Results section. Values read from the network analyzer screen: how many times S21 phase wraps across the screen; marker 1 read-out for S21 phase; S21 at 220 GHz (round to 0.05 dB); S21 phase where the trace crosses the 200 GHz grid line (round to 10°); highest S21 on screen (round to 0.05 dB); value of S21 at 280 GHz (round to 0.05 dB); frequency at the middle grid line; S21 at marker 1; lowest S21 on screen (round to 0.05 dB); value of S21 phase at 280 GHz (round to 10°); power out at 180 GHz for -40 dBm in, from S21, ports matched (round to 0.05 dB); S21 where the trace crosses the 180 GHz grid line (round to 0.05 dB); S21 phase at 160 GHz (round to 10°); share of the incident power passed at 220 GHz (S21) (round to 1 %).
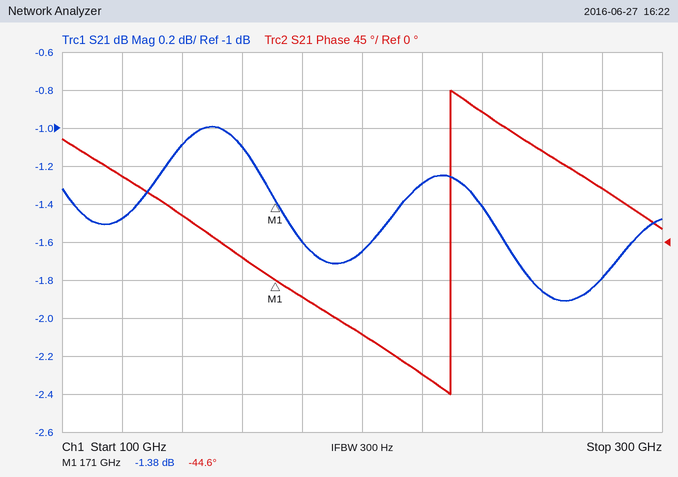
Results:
1
-44.6°
-1.30 dB
-110°
-1.00 dB
-1.80 dB
200 GHz
-1.38 dB
-1.90 dB
60°
-41.60 dBm
-1.60 dB
-20°
74 %
